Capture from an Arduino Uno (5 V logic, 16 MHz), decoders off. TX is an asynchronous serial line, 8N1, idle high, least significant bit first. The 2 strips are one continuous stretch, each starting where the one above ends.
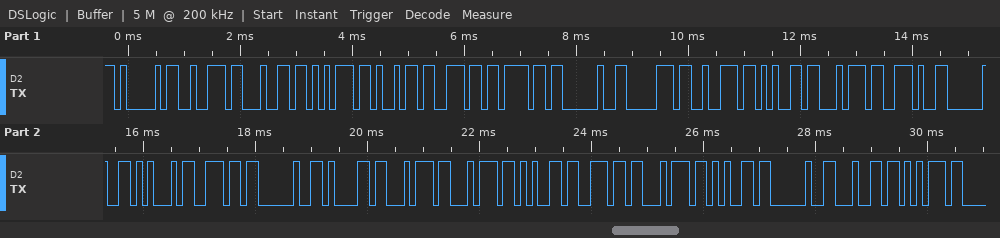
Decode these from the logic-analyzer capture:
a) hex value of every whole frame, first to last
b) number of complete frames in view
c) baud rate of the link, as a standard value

0x41 0x72 0x64 0x75 0x69 0x6E 0x6F 0x20 0x70 0x72 0x65 0x74 0x2E 0x20 0x45 0x6E 0x20 0x61 0x74 0x74 0x65 0x6E 0x74 0x65 0x20 0x64 0x75
27
9600 baud
